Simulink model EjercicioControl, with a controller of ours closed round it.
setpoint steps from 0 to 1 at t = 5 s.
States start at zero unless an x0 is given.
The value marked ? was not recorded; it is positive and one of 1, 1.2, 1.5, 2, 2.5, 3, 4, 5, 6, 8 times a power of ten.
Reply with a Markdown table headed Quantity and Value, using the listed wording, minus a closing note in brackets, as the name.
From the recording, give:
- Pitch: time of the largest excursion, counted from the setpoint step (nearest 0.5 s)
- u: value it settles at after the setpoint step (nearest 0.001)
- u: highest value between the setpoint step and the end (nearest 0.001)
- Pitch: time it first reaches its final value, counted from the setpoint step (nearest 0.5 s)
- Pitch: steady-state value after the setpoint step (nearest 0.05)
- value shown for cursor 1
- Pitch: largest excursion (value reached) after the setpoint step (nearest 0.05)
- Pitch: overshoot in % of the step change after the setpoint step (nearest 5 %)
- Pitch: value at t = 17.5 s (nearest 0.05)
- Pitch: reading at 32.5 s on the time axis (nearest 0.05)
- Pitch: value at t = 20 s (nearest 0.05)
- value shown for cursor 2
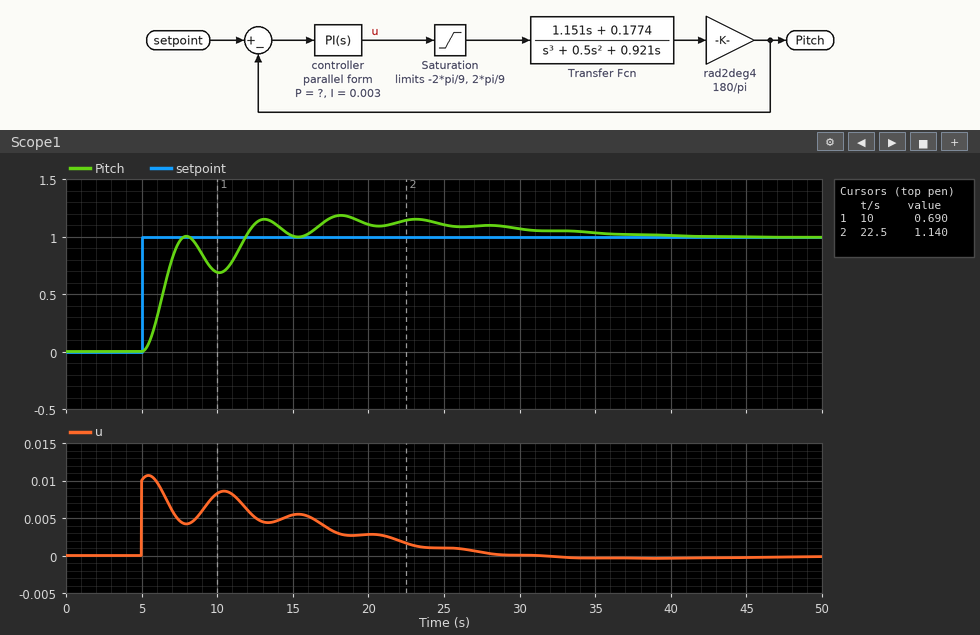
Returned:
| Quantity | Value |
|---|---|
| Pitch: time of the largest excursion, counted from the setpoint step | 13.0 s |
| u: value it settles at after the setpoint step | 0.000 |
| u: highest value between the setpoint step and the end | 0.011 |
| Pitch: time it first reaches its final value, counted from the setpoint step | 3.0 s |
| Pitch: steady-state value after the setpoint step | 1.00 |
| value shown for cursor 1 | 0.690 |
| Pitch: largest excursion (value reached) after the setpoint step | 1.20 |
| Pitch: overshoot in % of the step change after the setpoint step | 20 % |
| Pitch: value at t = 17.5 s | 1.15 |
| Pitch: reading at 32.5 s on the time axis | 1.05 |
| Pitch: value at t = 20 s | 1.10 |
| value shown for cursor 2 | 1.140 |
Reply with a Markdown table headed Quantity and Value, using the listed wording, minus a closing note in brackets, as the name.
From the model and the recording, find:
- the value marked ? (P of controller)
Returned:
| Quantity | Value |
|---|---|
| the value marked ? | 0.01 |
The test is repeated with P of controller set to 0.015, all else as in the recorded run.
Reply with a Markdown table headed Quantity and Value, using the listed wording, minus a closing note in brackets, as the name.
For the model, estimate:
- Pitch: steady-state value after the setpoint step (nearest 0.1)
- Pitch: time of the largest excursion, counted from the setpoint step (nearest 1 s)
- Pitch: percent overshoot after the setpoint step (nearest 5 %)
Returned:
| Quantity | Value |
|---|---|
| Pitch: steady-state value after the setpoint step | 1.0 |
| Pitch: time of the largest excursion, counted from the setpoint step | 12 s |
| Pitch: percent overshoot after the setpoint step | 15 % |
